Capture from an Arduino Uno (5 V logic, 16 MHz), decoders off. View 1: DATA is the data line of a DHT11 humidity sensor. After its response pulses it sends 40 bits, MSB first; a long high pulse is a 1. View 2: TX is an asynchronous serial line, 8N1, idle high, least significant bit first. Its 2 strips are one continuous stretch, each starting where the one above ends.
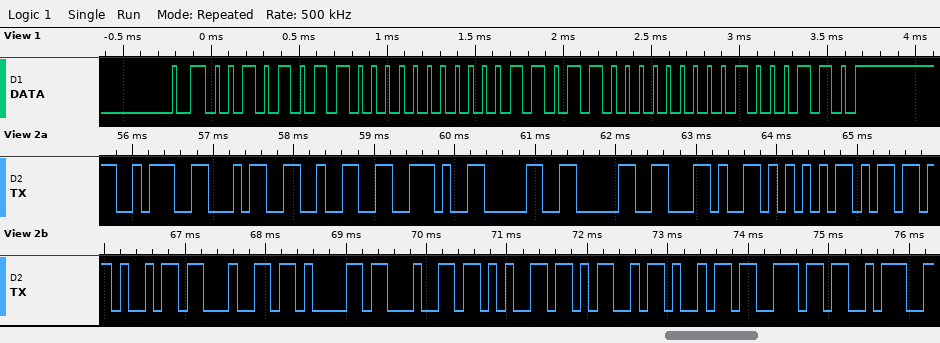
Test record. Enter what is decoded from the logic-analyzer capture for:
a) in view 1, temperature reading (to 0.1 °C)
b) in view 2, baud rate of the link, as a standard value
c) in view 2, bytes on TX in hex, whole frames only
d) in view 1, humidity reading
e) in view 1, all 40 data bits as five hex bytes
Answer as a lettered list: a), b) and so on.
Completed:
a) 27.0 °C
b) 9600 baud
c) 3A 34 32 2E 30 30 2C 55 6D 69 64 61 64 65 4D 69 6E 3A
d) 43 %
e) 2B 00 1B 00 46
